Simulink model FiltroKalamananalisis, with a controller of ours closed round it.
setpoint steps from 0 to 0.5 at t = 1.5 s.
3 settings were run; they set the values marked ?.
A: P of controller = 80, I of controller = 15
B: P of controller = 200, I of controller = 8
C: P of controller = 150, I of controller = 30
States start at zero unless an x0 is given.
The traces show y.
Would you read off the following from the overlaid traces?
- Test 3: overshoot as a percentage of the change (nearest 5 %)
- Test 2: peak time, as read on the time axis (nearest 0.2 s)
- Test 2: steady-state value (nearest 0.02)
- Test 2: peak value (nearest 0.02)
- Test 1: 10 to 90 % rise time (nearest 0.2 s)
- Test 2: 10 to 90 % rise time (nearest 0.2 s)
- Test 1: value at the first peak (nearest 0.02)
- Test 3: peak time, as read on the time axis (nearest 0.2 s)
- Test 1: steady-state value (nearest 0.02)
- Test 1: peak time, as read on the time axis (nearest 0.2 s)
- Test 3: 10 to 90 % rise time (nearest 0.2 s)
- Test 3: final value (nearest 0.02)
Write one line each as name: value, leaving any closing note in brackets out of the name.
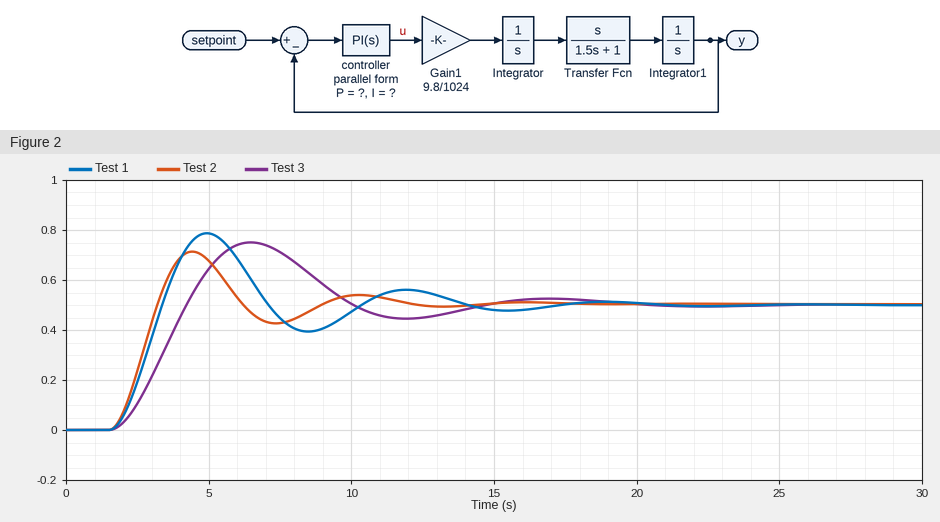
Test 3: overshoot as a percentage of the change: 50 %
Test 2: peak time, as read on the time axis: 4.4 s
Test 2: steady-state value: 0.50
Test 2: peak value: 0.72
Test 1: 10 to 90 % rise time: 1.2 s
Test 2: 10 to 90 % rise time: 1.2 s
Test 1: value at the first peak: 0.78
Test 3: peak time, as read on the time axis: 6.4 s
Test 1: steady-state value: 0.50
Test 1: peak time, as read on the time axis: 5.0 s
Test 3: 10 to 90 % rise time: 1.8 s
Test 3: final value: 0.50
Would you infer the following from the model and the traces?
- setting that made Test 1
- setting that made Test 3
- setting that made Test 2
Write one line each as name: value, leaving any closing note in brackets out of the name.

setting that made Test 1: C
setting that made Test 3: A
setting that made Test 2: B
